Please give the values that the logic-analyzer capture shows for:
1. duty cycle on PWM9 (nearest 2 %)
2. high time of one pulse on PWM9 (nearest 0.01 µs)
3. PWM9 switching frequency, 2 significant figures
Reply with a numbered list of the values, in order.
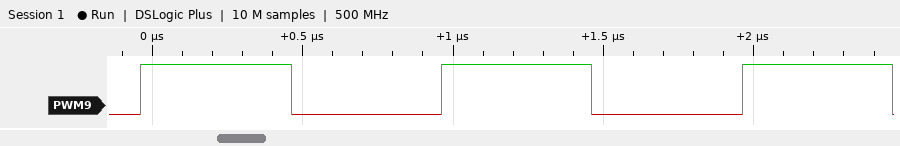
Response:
1. 50 %
2. 0.50 µs
3. 1.0 MHz
